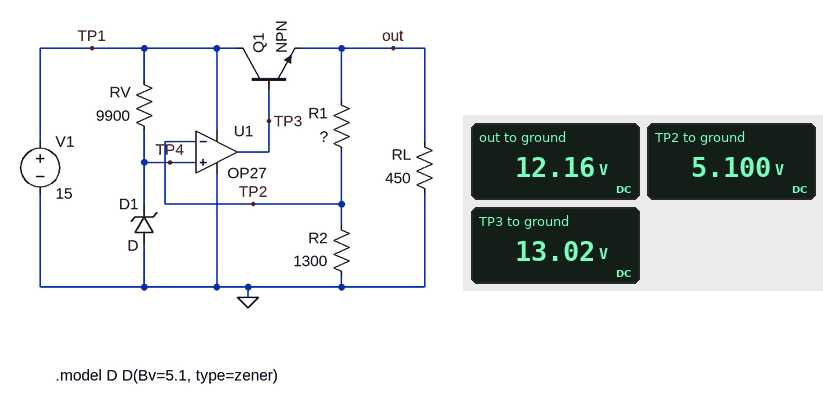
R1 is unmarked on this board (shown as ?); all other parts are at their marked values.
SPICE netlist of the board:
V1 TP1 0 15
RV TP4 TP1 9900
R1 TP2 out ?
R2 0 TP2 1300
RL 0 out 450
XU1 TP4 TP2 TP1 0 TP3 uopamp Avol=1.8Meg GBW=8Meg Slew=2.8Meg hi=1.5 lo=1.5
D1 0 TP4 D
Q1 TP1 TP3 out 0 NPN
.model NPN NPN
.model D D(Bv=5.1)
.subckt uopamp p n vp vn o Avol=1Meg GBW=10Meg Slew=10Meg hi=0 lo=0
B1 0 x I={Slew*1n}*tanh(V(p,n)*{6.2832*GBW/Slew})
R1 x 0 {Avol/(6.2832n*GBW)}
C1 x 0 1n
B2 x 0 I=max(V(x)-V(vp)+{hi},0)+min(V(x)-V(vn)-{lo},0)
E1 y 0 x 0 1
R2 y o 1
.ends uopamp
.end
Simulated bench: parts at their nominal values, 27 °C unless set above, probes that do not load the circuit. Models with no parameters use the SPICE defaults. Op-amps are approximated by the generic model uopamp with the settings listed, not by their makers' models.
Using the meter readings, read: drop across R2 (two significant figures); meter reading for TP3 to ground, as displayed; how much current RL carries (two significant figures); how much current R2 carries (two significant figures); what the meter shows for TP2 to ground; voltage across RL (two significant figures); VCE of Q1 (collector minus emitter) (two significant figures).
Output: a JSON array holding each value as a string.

["5.1 V", "13.02 V", "27 mA", "3.9 mA", "5.100 V", "12 V", "2.8 V"]
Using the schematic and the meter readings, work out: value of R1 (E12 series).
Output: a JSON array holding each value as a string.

["1.8 kΩ"]
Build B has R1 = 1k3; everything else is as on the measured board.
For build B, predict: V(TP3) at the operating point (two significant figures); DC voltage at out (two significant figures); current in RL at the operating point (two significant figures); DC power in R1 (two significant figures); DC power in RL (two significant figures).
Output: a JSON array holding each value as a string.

["11 V", "10 V", "23 mA", "20 mW", "230 mW"]
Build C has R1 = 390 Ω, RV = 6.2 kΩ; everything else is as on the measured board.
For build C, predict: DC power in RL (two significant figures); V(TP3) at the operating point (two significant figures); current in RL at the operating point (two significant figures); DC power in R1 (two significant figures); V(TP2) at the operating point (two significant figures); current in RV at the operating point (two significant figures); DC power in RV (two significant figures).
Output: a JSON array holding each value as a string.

["98 mW", "7.5 V", "15 mA", "6.0 mW", "5.1 V", "1.6 mA", "16 mW"]
